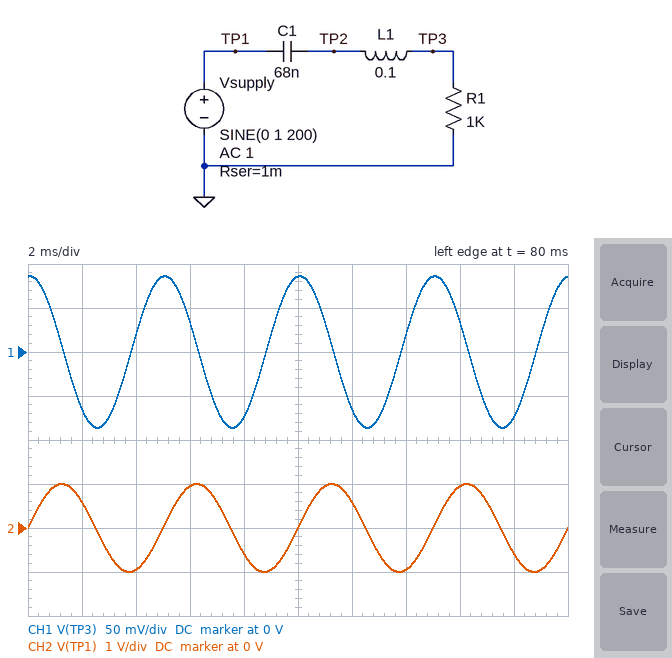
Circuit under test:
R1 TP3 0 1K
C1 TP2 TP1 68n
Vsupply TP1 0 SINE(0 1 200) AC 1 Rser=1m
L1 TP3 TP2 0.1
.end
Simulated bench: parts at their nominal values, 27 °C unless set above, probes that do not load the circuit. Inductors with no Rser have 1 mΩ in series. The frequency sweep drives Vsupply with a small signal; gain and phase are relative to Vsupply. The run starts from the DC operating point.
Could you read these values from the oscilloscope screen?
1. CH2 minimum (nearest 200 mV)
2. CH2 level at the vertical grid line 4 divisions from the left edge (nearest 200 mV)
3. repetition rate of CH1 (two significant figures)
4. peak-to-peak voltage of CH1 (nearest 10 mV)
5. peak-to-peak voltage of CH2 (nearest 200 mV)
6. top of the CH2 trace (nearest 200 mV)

-1.0 V
-600 mV
200 Hz
170 mV
2.0 V
1.0 V
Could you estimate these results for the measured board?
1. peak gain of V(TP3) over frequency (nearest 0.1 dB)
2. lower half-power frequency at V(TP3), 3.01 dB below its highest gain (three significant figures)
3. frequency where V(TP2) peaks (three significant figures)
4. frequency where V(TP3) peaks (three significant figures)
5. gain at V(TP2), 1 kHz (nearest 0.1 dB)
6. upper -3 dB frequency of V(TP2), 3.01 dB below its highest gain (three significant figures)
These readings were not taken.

0 dB
1.29 kHz
2.17 kHz
1.93 kHz
-4.5 dB
5.08 kHz
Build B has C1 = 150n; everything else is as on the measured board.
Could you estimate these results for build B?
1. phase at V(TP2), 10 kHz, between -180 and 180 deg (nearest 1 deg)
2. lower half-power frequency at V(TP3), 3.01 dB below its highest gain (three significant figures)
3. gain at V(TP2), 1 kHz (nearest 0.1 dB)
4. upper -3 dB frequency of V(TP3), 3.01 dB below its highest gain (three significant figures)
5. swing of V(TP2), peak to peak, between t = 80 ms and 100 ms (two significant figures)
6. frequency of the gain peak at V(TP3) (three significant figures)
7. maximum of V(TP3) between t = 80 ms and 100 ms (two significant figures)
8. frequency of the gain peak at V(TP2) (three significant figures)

0 deg
728 Hz
0.7 dB
2.32 kHz
380 mV
1.30 kHz
190 mV
1.59 kHz
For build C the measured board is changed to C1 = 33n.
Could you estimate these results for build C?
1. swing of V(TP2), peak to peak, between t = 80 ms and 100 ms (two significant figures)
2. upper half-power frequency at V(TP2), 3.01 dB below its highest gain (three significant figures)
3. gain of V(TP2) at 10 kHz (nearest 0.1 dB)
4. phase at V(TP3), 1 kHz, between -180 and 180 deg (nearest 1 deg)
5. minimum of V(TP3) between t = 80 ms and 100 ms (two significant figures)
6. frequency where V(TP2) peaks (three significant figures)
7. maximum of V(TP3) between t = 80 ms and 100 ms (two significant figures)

84 mV
4.62 kHz
0.7 dB
77 deg
-42 mV
2.96 kHz
42 mV
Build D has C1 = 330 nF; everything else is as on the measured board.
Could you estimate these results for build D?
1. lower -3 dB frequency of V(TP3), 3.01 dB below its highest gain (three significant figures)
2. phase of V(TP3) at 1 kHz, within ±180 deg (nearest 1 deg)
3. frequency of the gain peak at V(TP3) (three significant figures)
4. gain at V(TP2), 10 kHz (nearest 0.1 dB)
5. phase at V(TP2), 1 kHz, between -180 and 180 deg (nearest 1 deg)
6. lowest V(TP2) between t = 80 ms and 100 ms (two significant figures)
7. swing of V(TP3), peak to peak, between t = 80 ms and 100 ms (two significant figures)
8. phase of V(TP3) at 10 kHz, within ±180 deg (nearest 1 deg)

388 Hz
-8 deg
876 Hz
0.1 dB
24 deg
-400 mV
800 mV
-81 deg
